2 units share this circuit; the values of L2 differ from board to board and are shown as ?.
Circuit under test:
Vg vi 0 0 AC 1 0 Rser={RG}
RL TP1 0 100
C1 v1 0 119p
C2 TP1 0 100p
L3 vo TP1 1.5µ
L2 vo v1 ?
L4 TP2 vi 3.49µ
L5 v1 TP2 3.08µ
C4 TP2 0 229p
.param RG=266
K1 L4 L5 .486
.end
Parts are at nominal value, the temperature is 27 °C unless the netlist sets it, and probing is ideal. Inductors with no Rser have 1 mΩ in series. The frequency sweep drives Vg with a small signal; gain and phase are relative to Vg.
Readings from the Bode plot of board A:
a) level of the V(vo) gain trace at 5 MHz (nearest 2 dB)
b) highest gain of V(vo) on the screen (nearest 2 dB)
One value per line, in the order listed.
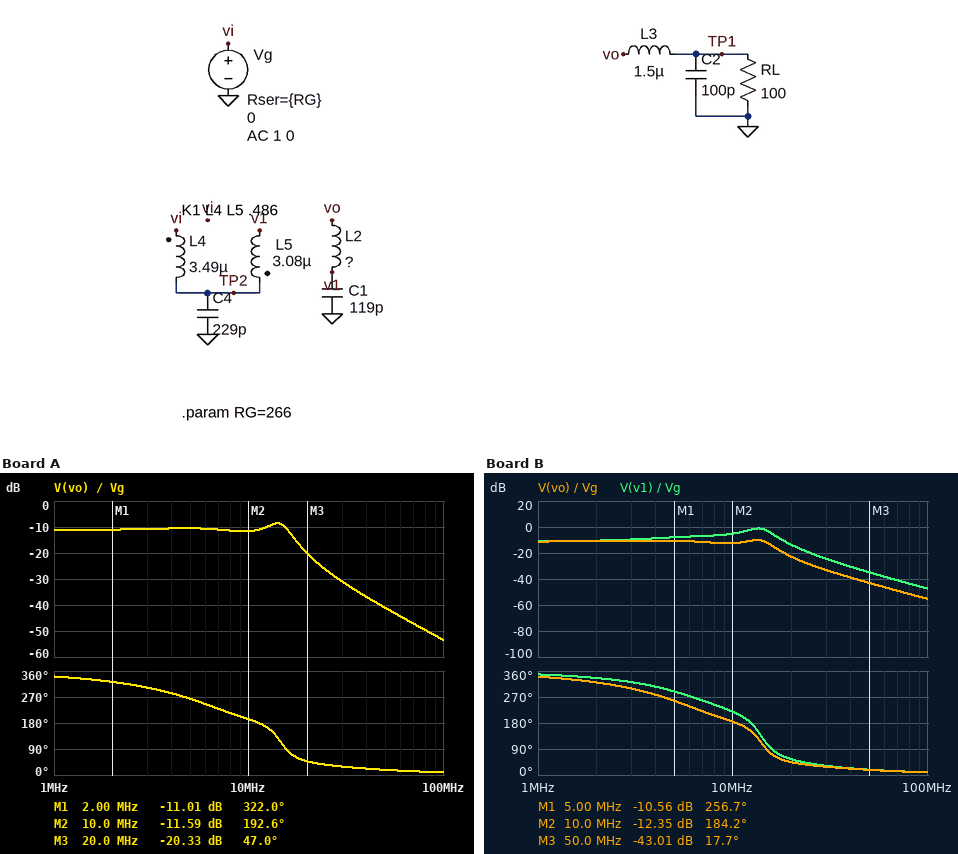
-10 dB
-8 dB
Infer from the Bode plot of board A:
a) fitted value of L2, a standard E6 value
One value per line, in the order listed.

1.5 µH
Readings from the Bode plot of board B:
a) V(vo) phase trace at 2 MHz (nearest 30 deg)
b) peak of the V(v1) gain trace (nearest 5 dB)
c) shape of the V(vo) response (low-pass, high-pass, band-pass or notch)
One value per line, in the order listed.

330 deg
0 dB
low-pass
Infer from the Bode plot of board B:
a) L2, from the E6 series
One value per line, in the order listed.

2.2 µH
